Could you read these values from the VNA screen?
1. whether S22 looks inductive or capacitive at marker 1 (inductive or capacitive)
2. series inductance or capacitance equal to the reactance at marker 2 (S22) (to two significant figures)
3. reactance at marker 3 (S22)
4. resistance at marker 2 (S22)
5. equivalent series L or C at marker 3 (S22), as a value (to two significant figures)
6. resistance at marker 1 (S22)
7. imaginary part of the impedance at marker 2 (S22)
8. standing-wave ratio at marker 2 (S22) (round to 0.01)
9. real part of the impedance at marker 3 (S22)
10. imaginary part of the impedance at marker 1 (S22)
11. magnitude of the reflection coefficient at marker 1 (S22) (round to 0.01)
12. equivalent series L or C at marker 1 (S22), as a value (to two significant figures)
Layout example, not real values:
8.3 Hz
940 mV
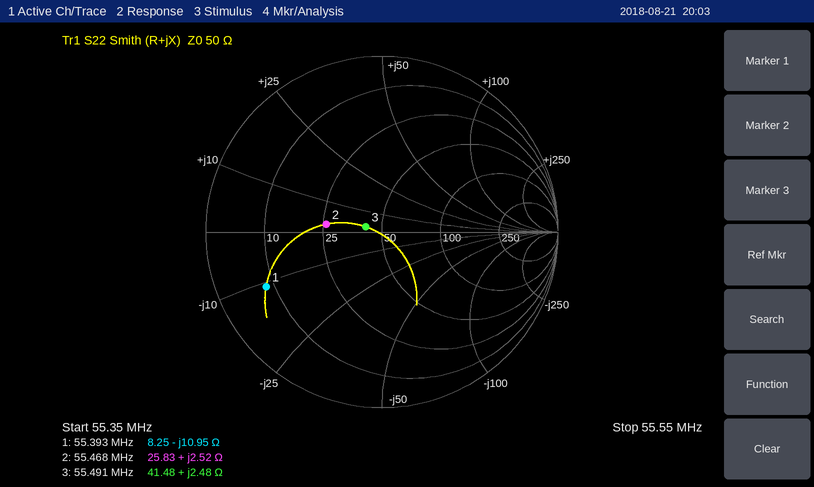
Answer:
capacitive
7.2 nH
+2.48 Ω
25.83 Ω
7.1 nH
8.25 Ω
+2.52 Ω
1.94
41.48 Ω
-10.95 Ω
0.73
260 pF
